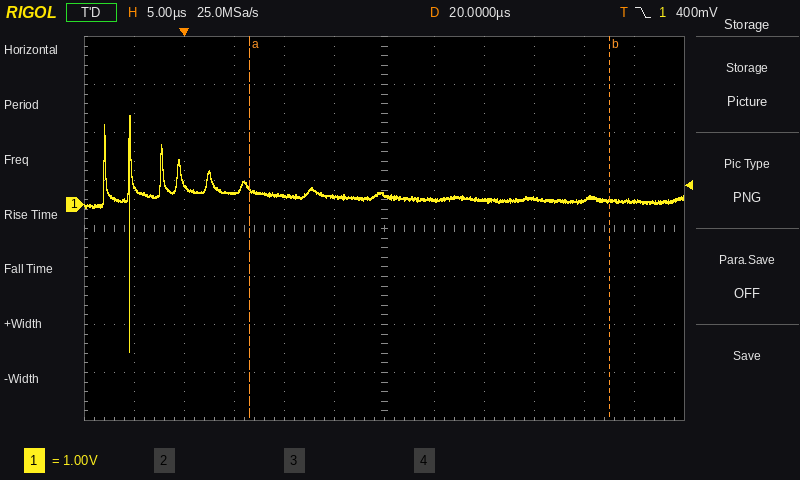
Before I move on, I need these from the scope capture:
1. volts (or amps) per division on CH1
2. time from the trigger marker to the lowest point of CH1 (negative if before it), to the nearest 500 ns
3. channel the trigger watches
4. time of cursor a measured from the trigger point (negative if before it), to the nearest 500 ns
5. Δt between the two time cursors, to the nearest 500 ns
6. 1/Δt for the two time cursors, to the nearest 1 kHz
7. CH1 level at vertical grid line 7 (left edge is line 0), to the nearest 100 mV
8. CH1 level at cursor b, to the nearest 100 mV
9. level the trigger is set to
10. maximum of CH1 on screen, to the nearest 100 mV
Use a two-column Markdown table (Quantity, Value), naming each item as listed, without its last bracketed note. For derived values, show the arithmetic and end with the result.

| Quantity | Value |
|---|---|
| volts (or amps) per division on CH1 | 1 V |
| time from the trigger marker to the lowest point of CH1 (negative if before it), to the nearest 500 ns | -5.5 µs |
| channel the trigger watches | CH1 |
| time of cursor a measured from the trigger point (negative if before it), to the nearest 500 ns | +6.5 µs |
| Δt between the two time cursors, to the nearest 500 ns | 36.0 µs |
| 1/Δt for the two time cursors, to the nearest 1 kHz | 1 / 36.0 µs ≈ 28 kHz |
| CH1 level at vertical grid line 7 (left edge is line 0), to the nearest 100 mV | 100 mV |
| CH1 level at cursor b, to the nearest 100 mV | 100 mV |
| level the trigger is set to | 400 mV |
| maximum of CH1 on screen, to the nearest 100 mV | 1.9 V |
